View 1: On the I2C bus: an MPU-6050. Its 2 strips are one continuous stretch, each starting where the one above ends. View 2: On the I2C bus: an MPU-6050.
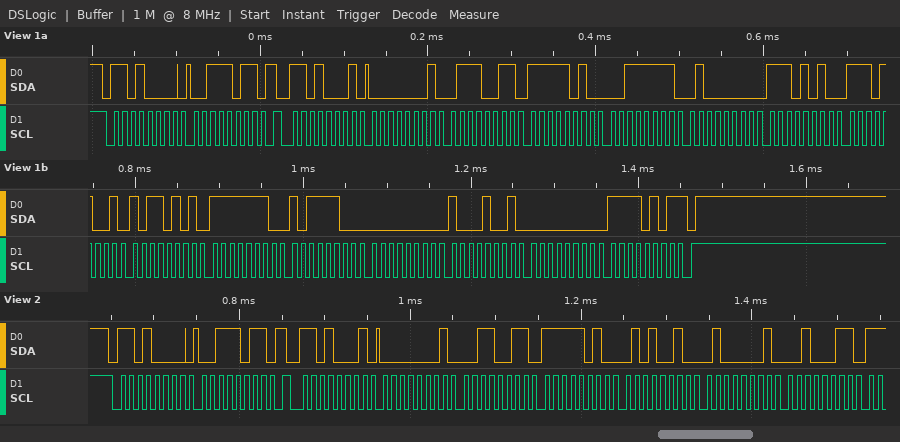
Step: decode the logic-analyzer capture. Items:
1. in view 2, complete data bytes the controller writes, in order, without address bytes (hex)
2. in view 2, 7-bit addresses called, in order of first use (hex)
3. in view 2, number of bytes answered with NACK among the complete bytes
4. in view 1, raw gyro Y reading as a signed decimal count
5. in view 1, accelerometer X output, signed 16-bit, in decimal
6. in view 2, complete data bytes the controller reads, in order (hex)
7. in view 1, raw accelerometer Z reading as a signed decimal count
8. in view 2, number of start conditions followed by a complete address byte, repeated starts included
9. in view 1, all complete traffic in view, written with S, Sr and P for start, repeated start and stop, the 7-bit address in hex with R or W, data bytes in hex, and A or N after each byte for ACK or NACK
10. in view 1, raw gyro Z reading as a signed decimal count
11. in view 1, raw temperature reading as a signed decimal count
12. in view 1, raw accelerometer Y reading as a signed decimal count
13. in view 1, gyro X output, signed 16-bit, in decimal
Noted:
3B
0x68
0
137
371
01 33 FA 52 41 23
16618
2
S 68W A 3B A Sr 68R A 01 A 73 A FA A 3F A 40 A EA A E9 A B5 A FE A BC A 00 A 89 A 00 A F5 N P
245
-5707
-1473
-324
